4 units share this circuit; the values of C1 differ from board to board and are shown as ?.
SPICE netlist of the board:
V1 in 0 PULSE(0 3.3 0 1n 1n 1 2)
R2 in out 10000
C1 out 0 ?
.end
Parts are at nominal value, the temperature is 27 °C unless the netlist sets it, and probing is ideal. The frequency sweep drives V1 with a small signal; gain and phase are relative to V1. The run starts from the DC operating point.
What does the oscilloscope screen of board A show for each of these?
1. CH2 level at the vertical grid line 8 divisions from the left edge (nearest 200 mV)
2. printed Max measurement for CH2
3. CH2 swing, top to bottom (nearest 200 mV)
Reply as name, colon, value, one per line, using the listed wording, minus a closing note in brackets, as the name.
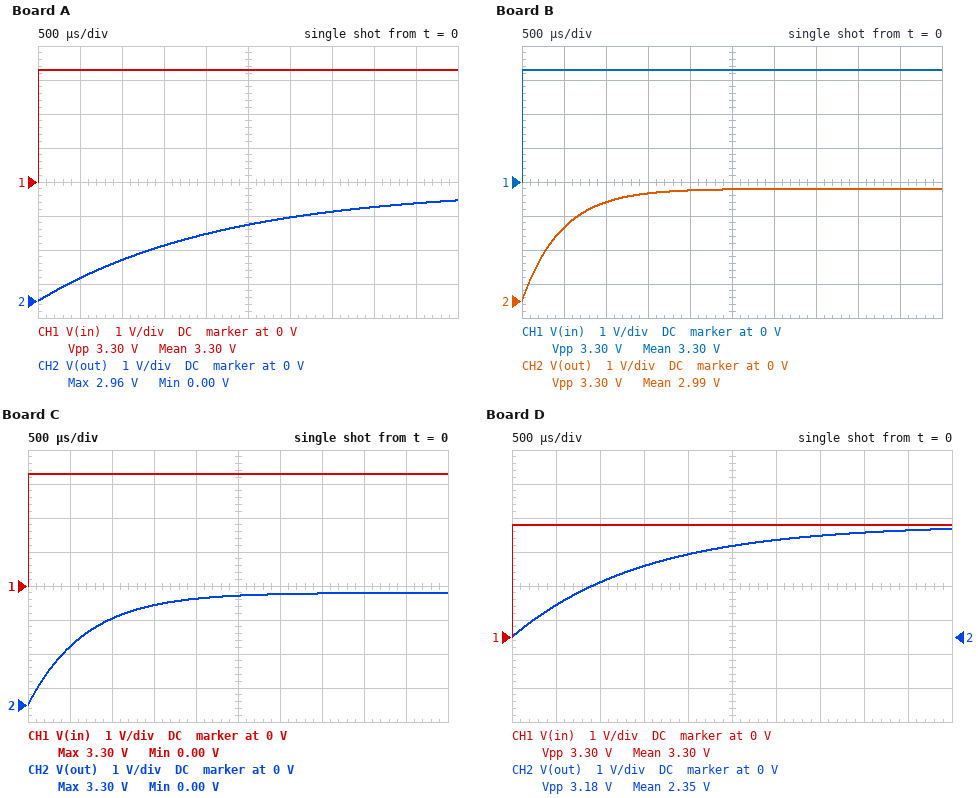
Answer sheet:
CH2 level at the vertical grid line 8 divisions from the left edge: 2.8 V
printed Max measurement for CH2: 2.96 V
CH2 swing, top to bottom: 3.0 V
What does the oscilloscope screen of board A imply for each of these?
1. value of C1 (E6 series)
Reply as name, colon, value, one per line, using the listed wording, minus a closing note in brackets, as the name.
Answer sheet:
value of C1: 220 nF
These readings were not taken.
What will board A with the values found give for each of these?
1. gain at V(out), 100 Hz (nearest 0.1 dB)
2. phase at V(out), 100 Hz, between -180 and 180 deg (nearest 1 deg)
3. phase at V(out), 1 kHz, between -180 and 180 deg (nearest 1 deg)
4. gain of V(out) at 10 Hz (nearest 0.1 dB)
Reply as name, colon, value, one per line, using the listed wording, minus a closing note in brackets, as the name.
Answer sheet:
gain at V(out), 100 Hz: -4.6 dB
phase at V(out), 100 Hz, between -180 and 180 deg: -54 deg
phase at V(out), 1 kHz, between -180 and 180 deg: -86 deg
gain of V(out) at 10 Hz: -0.1 dB
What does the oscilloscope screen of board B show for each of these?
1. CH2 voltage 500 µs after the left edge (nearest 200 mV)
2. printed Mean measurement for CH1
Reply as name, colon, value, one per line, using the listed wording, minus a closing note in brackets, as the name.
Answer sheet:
CH2 voltage 500 µs after the left edge: 2.2 V
printed Mean measurement for CH1: 3.30 V
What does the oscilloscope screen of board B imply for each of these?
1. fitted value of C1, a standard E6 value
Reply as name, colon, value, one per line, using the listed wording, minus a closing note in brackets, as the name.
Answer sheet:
fitted value of C1, a standard E6 value: 47 nF
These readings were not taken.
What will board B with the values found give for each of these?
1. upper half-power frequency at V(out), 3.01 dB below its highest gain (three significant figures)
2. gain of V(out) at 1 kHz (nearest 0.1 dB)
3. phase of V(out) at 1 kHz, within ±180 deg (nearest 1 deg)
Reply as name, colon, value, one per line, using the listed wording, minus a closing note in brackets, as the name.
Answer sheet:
upper half-power frequency at V(out), 3.01 dB below its highest gain: 339 Hz
gain of V(out) at 1 kHz: -9.9 dB
phase of V(out) at 1 kHz, within ±180 deg: -71 deg
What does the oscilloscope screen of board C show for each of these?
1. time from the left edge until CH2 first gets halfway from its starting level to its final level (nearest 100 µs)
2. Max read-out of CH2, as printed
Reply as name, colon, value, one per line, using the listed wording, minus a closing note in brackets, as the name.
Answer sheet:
time from the left edge until CH2 first gets halfway from its starting level to its final level: 500 µs
Max read-out of CH2, as printed: 3.30 V
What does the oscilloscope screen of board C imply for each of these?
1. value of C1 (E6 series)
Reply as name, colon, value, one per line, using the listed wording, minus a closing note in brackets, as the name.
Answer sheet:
value of C1: 68 nF
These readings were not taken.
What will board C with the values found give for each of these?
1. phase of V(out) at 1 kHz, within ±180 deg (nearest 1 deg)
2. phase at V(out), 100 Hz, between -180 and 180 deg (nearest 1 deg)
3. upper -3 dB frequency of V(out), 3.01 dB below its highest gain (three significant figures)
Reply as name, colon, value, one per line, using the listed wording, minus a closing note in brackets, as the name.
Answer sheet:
phase of V(out) at 1 kHz, within ±180 deg: -77 deg
phase at V(out), 100 Hz, between -180 and 180 deg: -23 deg
upper -3 dB frequency of V(out), 3.01 dB below its highest gain: 234 Hz
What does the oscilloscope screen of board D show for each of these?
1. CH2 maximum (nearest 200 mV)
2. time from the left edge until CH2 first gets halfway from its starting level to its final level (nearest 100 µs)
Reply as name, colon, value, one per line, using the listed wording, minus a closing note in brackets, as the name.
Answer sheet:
CH2 maximum: 3.2 V
time from the left edge until CH2 first gets halfway from its starting level to its final level: 1.0 ms
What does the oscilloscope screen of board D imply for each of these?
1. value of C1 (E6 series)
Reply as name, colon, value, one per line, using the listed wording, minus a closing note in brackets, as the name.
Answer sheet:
value of C1: 150 nF
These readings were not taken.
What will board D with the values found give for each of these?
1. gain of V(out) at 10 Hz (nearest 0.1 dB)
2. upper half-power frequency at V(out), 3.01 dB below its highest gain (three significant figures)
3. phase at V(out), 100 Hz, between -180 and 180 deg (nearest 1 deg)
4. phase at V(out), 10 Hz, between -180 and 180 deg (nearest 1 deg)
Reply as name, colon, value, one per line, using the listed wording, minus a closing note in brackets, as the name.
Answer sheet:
gain of V(out) at 10 Hz: 0 dB
upper half-power frequency at V(out), 3.01 dB below its highest gain: 106 Hz
phase at V(out), 100 Hz, between -180 and 180 deg: -43 deg
phase at V(out), 10 Hz, between -180 and 180 deg: -5 deg
